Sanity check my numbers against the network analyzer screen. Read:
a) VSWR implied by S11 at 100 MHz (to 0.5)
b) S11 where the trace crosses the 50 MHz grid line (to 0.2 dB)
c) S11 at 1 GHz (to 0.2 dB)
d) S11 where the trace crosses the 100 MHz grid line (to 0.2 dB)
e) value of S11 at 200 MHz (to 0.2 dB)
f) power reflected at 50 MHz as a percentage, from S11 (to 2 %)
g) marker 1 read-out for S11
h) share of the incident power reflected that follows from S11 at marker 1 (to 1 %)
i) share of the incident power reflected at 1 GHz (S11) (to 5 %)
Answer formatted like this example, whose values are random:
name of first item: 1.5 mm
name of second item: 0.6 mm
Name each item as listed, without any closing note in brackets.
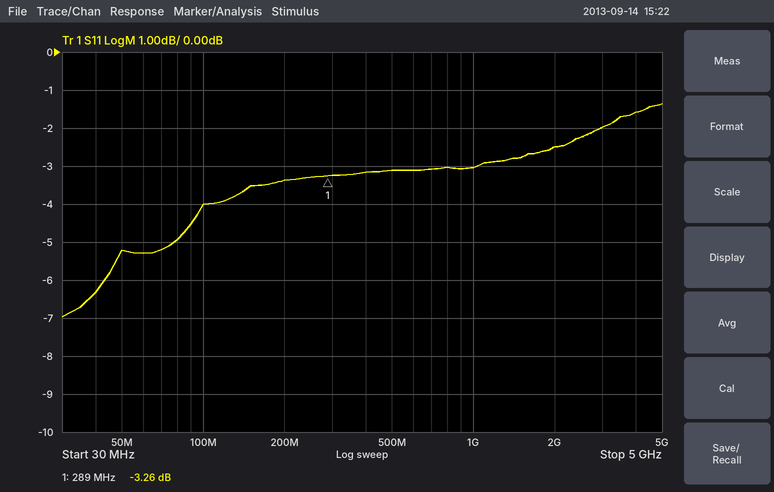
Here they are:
VSWR implied by S11 at 100 MHz: 4.5
S11 where the trace crosses the 50 MHz grid line: -5.2 dB
S11 at 1 GHz: -3.0 dB
S11 where the trace crosses the 100 MHz grid line: -4.0 dB
value of S11 at 200 MHz: -3.4 dB
power reflected at 50 MHz as a percentage, from S11: 30 %
marker 1 read-out for S11: -3.26 dB
share of the incident power reflected that follows from S11 at marker 1: 47 %
share of the incident power reflected at 1 GHz (S11): 50 %
